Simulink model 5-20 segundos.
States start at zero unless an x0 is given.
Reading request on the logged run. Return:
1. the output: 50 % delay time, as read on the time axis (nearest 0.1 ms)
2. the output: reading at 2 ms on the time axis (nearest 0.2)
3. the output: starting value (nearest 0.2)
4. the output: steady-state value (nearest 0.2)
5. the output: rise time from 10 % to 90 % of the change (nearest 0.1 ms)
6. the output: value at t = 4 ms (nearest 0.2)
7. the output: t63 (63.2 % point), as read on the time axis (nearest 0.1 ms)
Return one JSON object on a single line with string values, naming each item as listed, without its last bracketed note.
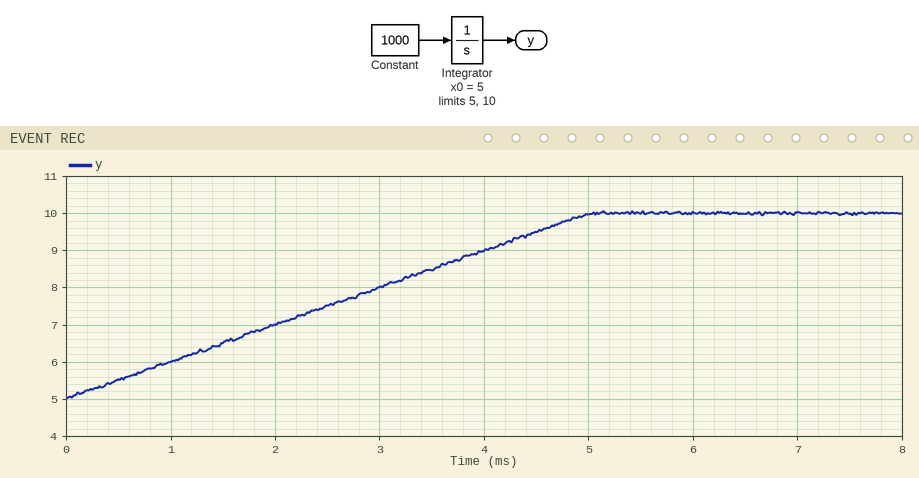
{"the output: 50 % delay time, as read on the time axis": "2.5 ms", "the output: reading at 2 ms on the time axis": "7.0", "the output: starting value": "5.0", "the output: steady-state value": "10.0", "the output: rise time from 10 % to 90 % of the change": "4.0 ms", "the output: value at t = 4 ms": "9.0", "the output: t63 (63.2 % point), as read on the time axis": "3.2 ms"}
